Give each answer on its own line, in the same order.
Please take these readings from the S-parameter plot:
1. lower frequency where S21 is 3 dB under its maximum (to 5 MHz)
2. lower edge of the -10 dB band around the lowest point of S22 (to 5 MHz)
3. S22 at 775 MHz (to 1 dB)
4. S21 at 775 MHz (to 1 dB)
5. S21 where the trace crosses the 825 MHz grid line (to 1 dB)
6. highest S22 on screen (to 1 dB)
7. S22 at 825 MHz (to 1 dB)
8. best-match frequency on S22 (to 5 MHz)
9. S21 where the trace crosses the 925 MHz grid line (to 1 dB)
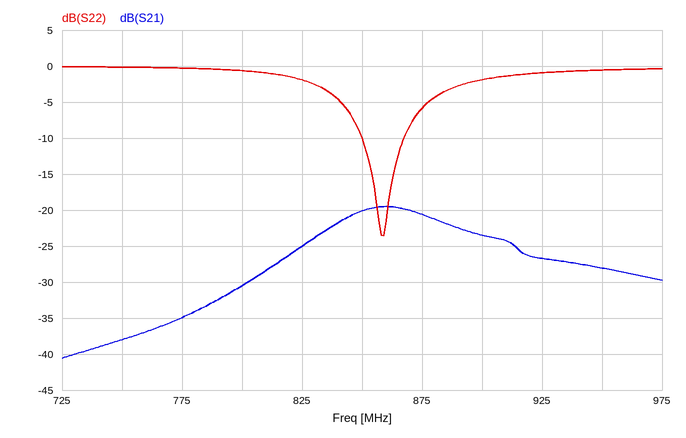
835 MHz
850 MHz
0 dB
-35 dB
-25 dB
0 dB
-2 dB
860 MHz
-27 dB
